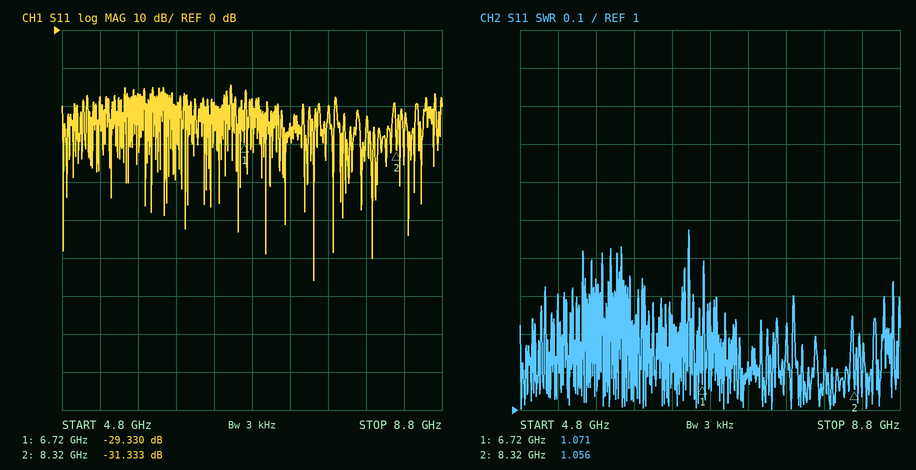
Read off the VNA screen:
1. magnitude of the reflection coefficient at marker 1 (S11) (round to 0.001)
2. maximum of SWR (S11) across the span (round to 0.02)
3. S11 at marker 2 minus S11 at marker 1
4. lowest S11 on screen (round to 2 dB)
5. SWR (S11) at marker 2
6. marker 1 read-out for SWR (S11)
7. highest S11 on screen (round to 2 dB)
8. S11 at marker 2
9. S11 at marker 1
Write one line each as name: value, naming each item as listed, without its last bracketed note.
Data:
magnitude of the reflection coefficient at marker 1 (S11): 0.034
maximum of SWR (S11) across the span: 1.48
S11 at marker 2 minus S11 at marker 1: -2.003 dB
lowest S11 on screen: -66 dB
SWR (S11) at marker 2: 1.056
marker 1 read-out for SWR: 1.071
highest S11 on screen: -14 dB
S11 at marker 2: -31.333 dB
S11 at marker 1: -29.330 dB
